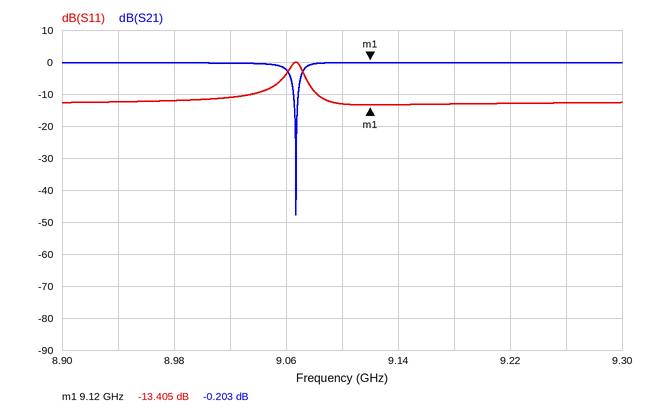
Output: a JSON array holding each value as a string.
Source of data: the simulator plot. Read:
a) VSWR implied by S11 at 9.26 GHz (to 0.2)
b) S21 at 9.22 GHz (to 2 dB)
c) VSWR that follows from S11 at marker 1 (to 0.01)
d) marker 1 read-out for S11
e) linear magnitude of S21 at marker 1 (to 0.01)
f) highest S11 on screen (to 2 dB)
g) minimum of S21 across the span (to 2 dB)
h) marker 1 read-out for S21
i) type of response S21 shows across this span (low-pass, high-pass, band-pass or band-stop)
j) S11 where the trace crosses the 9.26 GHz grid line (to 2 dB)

["1.6", "0 dB", "1.54", "-13.405 dB", "0.98", "0 dB", "-48 dB", "-0.203 dB", "band-stop", "-12 dB"]
